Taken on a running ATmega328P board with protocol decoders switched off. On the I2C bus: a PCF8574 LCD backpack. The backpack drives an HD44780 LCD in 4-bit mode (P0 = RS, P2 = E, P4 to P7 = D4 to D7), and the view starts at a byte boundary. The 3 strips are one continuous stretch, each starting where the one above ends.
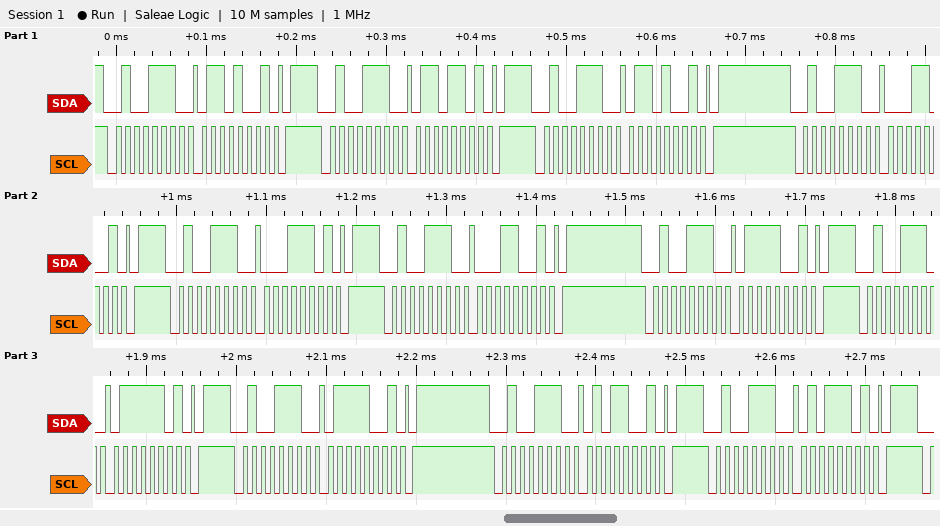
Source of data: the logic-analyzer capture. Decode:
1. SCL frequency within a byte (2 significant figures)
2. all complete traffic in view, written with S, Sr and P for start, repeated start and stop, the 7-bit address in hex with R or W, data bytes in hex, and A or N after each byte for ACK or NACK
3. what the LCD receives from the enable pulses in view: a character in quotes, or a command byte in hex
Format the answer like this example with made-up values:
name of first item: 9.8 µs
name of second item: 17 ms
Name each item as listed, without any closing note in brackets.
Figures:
SCL frequency within a byte: 100 kHz
all complete traffic in view, written with S, Sr and P for start, repeated start and stop, the 7-bit address in hex with R or W, data bytes in hex, and A or N after each byte for ACK or NACK: S 27W A 69 A P S 27W A 6D A P S 27W A 69 A P S 27W A 19 A P S 27W A 1D A P S 27W A 19 A P S 27W A 79 A P S 27W A 7D A P S 27W A 79 A P S 27W A 59 A P S 27W A 5D A P
what the LCD receives from the enable pulses in view: a character in quotes, or a command byte in hex: 'a'
